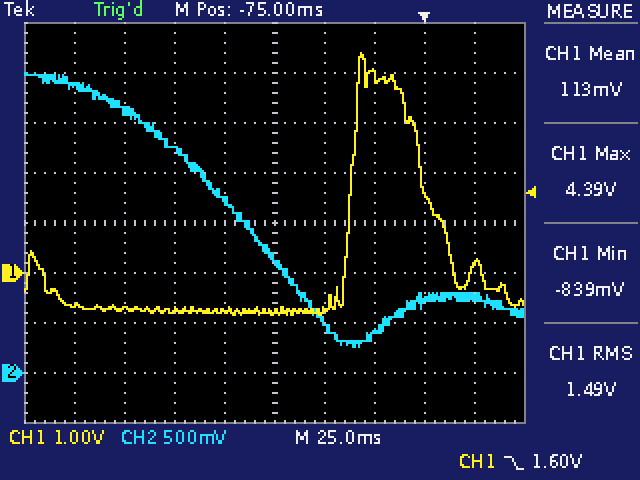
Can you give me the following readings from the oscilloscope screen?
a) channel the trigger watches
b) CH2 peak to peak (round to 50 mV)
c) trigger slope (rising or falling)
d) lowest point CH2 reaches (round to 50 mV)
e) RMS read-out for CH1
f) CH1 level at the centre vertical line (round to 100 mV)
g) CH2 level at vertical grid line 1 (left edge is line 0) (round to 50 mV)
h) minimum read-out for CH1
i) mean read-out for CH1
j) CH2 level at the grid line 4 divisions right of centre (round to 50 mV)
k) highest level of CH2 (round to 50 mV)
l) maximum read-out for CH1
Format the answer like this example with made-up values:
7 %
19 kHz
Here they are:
CH1
2.75 V
falling
250 mV
1.49 V
-800 mV
2.85 V
-839 mV
113 mV
750 mV
3.00 V
4.39 V
